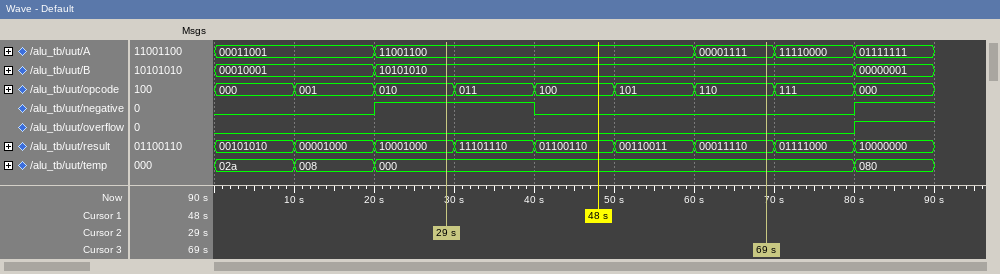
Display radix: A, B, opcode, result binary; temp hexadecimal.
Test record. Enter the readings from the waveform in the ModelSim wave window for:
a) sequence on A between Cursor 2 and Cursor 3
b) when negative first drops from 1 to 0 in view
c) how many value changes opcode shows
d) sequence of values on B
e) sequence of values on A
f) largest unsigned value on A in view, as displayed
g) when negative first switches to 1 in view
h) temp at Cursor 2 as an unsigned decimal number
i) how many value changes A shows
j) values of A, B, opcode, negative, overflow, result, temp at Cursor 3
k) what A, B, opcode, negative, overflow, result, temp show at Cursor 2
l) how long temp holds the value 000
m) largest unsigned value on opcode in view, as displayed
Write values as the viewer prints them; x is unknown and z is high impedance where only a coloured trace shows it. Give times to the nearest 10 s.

11001100, 00001111
40 s
8
00010001, 10101010, 00000001
00011001, 11001100, 00001111, 11110000, 01111111
11110000
20 s
0
4
A=00001111, B=10101010, opcode=110, negative=0, overflow=0, result=00011110, temp=000
A=11001100, B=10101010, opcode=010, negative=1, overflow=0, result=10001000, temp=000
60 s
111
